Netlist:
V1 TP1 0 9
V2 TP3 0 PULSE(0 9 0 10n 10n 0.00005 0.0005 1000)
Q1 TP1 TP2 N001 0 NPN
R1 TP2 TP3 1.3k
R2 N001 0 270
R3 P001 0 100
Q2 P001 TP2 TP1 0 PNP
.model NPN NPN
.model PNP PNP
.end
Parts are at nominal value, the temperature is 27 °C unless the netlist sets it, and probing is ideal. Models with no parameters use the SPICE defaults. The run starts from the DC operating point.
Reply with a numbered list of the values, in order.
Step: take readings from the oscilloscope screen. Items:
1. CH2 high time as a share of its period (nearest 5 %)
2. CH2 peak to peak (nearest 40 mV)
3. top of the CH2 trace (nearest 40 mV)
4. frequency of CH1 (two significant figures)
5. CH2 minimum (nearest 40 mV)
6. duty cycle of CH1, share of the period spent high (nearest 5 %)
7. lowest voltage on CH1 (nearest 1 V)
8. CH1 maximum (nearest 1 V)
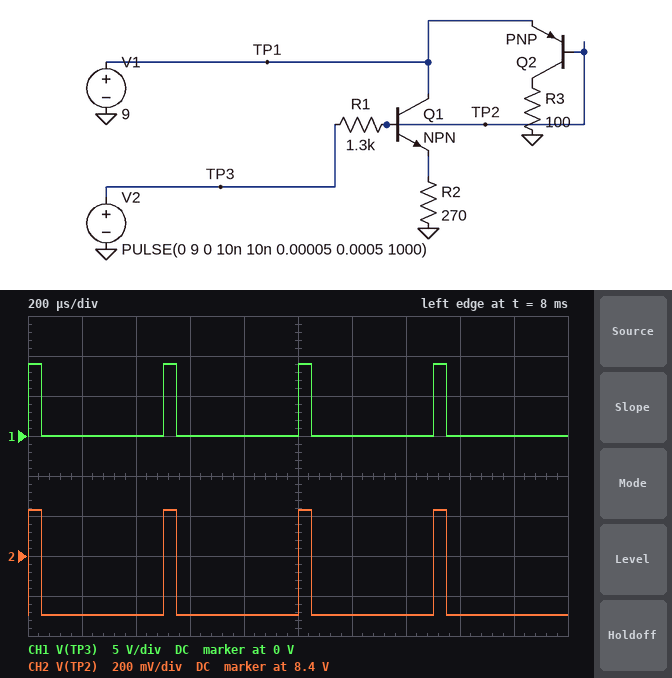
1. 10 %
2. 520 mV
3. 8.64 V
4. 2.0 kHz
5. 8.12 V
6. 10 %
7. 0 V
8. 9 V
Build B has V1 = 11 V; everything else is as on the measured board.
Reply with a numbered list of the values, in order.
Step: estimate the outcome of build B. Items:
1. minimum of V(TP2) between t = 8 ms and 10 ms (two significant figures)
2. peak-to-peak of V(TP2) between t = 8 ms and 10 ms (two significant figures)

1. 10 V
2. 3.3 mV
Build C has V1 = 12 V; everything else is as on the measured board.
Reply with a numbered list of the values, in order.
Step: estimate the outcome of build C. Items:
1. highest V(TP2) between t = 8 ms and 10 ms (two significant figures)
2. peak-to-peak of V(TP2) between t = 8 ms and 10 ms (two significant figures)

1. 11 V
2. 2.9 mV
